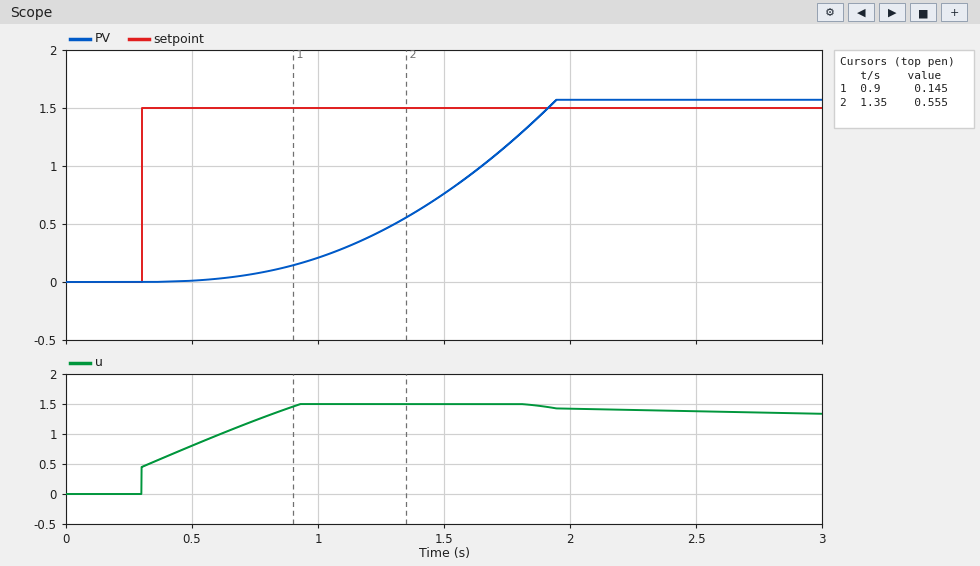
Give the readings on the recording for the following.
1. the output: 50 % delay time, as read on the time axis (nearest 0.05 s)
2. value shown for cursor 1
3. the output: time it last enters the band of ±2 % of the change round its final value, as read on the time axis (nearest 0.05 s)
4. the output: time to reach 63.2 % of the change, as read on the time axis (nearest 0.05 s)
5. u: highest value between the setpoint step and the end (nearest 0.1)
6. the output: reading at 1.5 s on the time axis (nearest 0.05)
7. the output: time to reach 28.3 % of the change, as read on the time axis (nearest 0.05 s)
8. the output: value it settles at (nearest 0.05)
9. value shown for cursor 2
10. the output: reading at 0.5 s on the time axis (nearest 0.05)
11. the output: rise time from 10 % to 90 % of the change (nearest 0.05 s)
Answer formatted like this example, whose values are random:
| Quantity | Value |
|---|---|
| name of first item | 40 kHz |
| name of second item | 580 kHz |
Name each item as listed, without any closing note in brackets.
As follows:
| Quantity | Value |
|---|---|
| the output: 50 % delay time, as read on the time axis | 1.50 s |
| value shown for cursor 1 | 0.145 |
| the output: time it last enters the band of ±2 % of the change round its final value, as read on the time axis | 1.95 s |
| the output: time to reach 63.2 % of the change, as read on the time axis | 1.65 s |
| u: highest value between the setpoint step and the end | 1.5 |
| the output: reading at 1.5 s on the time axis | 0.75 |
| the output: time to reach 28.3 % of the change, as read on the time axis | 1.25 s |
| the output: value it settles at | 1.55 |
| value shown for cursor 2 | 0.555 |
| the output: reading at 0.5 s on the time axis | 0.00 |
| the output: rise time from 10 % to 90 % of the change | 0.95 s |
